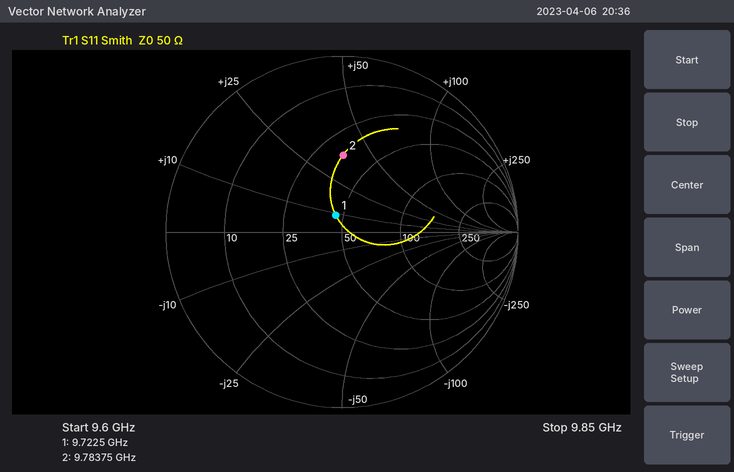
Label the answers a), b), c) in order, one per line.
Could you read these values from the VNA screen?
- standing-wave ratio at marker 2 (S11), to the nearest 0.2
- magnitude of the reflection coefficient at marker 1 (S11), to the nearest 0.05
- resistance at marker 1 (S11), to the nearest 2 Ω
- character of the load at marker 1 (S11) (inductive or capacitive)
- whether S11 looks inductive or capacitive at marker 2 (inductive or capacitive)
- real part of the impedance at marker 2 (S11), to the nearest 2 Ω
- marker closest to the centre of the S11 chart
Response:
a) 2.6
b) 0.10
c) 46 Ω
d) inductive
e) inductive
f) 34 Ω
g) marker 1
